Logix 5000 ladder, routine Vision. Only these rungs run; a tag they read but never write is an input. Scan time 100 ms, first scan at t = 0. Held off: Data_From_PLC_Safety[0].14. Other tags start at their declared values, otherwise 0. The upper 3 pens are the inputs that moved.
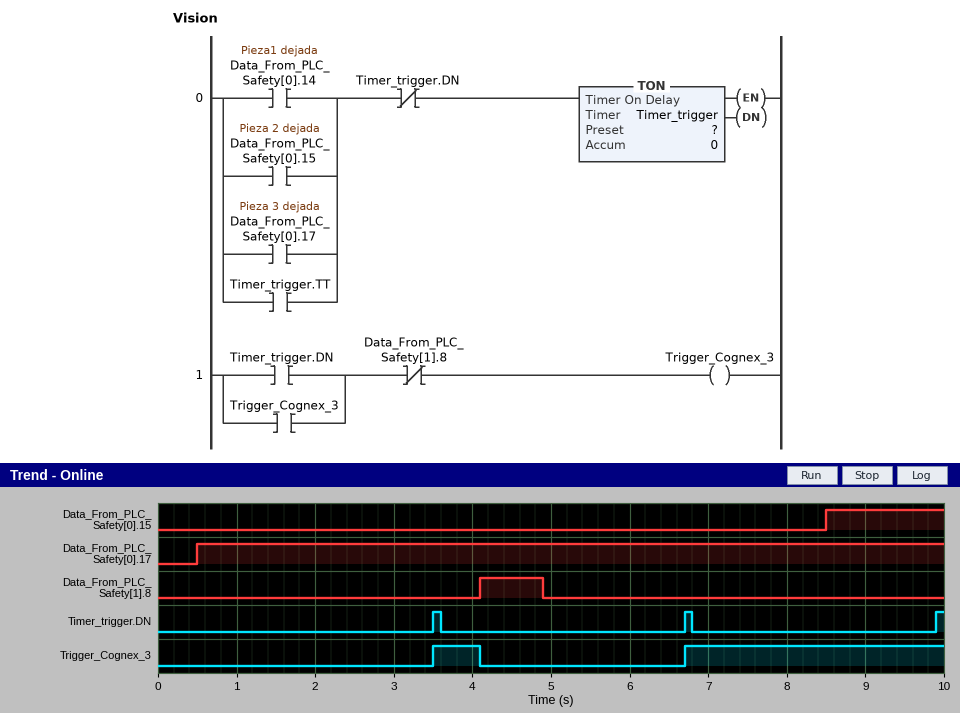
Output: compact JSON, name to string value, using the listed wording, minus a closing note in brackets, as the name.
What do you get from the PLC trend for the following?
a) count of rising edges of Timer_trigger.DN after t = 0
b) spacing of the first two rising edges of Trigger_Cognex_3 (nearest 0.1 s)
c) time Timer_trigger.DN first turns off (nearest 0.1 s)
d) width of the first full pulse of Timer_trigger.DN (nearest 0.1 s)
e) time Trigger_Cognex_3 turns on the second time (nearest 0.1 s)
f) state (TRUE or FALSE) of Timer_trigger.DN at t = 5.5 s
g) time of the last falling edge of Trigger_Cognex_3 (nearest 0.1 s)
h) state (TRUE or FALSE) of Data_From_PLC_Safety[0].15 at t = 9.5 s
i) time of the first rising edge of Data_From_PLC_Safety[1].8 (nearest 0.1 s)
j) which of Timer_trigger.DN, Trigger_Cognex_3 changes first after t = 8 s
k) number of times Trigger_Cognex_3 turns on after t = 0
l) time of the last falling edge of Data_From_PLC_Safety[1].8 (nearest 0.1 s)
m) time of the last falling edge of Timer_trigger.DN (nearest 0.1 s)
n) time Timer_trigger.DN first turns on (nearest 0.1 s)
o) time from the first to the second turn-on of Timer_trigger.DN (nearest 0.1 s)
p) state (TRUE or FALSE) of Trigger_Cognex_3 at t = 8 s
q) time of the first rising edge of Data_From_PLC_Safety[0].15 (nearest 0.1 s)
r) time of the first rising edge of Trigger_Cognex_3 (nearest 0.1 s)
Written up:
{"count of rising edges of Timer_trigger.DN after t = 0": "3", "spacing of the first two rising edges of Trigger_Cognex_3": "3.2 s", "time Timer_trigger.DN first turns off": "3.6 s", "width of the first full pulse of Timer_trigger.DN": "0.1 s", "time Trigger_Cognex_3 turns on the second time": "6.7 s", "state (TRUE or FALSE) of Timer_trigger.DN at t = 5.5 s": "FALSE", "time of the last falling edge of Trigger_Cognex_3": "4.1 s", "state (TRUE or FALSE) of Data_From_PLC_Safety[0].15 at t = 9.5 s": "TRUE", "time of the first rising edge of Data_From_PLC_Safety[1].8": "4.1 s", "which of Timer_trigger.DN, Trigger_Cognex_3 changes first after t = 8 s": "Timer_trigger.DN", "number of times Trigger_Cognex_3 turns on after t = 0": "2", "time of the last falling edge of Data_From_PLC_Safety[1].8": "4.9 s", "time of the last falling edge of Timer_trigger.DN": "6.8 s", "time Timer_trigger.DN first turns on": "3.5 s", "time from the first to the second turn-on of Timer_trigger.DN": "3.2 s", "state (TRUE or FALSE) of Trigger_Cognex_3 at t = 8 s": "TRUE", "time of the first rising edge of Data_From_PLC_Safety[0].15": "8.5 s", "time of the first rising edge of Trigger_Cognex_3": "3.5 s"}
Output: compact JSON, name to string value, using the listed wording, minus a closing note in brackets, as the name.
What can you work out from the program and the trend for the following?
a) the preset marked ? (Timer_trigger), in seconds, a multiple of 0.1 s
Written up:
{"the preset marked ? (Timer_trigger), in seconds, a multiple of 0.1 s": "3.0 s"}
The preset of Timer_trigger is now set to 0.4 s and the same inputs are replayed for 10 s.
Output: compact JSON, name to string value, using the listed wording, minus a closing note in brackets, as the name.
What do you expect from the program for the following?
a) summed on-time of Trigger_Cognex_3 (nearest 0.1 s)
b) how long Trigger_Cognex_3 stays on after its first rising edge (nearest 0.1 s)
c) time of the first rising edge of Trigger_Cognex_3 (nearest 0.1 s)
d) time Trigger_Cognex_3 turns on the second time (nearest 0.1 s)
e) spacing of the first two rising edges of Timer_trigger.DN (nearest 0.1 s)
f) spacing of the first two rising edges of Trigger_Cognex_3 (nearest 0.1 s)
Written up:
{"summed on-time of Trigger_Cognex_3": "8.1 s", "how long Trigger_Cognex_3 stays on after its first rising edge": "3.2 s", "time of the first rising edge of Trigger_Cognex_3": "0.9 s", "time Trigger_Cognex_3 turns on the second time": "5.1 s", "spacing of the first two rising edges of Timer_trigger.DN": "0.6 s", "spacing of the first two rising edges of Trigger_Cognex_3": "4.2 s"}
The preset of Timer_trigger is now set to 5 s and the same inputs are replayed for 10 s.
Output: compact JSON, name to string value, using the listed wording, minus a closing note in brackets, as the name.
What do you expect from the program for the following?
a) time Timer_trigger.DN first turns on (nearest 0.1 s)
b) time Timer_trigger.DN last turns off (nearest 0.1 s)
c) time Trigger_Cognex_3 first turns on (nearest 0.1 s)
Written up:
{"time Timer_trigger.DN first turns on": "5.5 s", "time Timer_trigger.DN last turns off": "5.6 s", "time Trigger_Cognex_3 first turns on": "5.5 s"}
